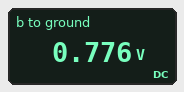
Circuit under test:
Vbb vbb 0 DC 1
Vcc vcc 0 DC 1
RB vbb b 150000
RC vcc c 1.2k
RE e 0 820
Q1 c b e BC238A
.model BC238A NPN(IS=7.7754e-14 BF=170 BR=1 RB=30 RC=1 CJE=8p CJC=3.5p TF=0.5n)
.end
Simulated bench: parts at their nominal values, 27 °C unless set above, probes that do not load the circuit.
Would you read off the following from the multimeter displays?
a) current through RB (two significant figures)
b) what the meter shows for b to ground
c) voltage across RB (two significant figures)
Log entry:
1.5 µA
0.776 V
220 mV
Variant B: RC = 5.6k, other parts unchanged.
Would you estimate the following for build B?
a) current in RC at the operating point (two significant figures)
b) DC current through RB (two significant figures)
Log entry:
140 µA
2.2 µA
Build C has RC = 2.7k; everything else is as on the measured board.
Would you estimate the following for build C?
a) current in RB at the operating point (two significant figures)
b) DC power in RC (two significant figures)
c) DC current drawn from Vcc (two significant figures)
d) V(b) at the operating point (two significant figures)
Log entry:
1.6 µA
150 µW
230 µA
760 mV
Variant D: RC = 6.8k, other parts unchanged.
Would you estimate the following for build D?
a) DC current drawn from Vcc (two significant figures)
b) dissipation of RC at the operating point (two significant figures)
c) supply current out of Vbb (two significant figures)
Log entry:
120 µA
92 µW
2.4 µA
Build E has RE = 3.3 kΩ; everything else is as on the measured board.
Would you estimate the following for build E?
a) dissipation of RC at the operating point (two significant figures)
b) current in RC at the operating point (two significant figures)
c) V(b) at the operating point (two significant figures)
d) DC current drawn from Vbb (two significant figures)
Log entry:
14 µW
110 µA
900 mV
640 nA
